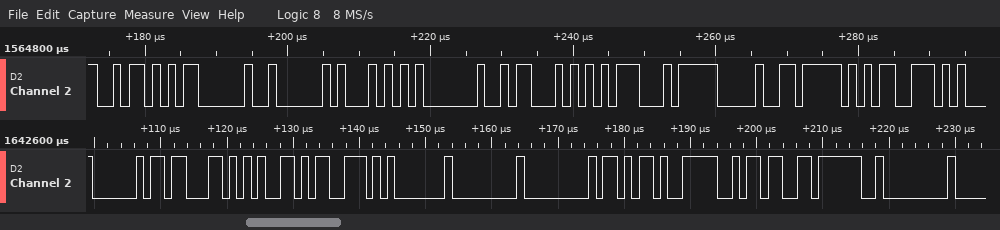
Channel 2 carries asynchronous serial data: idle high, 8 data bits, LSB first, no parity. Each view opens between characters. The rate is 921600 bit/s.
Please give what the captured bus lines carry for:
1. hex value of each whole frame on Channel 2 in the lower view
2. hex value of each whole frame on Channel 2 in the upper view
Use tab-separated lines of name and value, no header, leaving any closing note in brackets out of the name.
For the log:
hex value of each whole frame on Channel 2 in the lower view	A0, 63, 65, 73, 01, 00, 00, 6B, 3E, 9B, 3F, 00
hex value of each whole frame on Channel 2 in the upper view	5A, 03, 02, 51, 01, 1A, D5, F4, 90, 5F, 73
